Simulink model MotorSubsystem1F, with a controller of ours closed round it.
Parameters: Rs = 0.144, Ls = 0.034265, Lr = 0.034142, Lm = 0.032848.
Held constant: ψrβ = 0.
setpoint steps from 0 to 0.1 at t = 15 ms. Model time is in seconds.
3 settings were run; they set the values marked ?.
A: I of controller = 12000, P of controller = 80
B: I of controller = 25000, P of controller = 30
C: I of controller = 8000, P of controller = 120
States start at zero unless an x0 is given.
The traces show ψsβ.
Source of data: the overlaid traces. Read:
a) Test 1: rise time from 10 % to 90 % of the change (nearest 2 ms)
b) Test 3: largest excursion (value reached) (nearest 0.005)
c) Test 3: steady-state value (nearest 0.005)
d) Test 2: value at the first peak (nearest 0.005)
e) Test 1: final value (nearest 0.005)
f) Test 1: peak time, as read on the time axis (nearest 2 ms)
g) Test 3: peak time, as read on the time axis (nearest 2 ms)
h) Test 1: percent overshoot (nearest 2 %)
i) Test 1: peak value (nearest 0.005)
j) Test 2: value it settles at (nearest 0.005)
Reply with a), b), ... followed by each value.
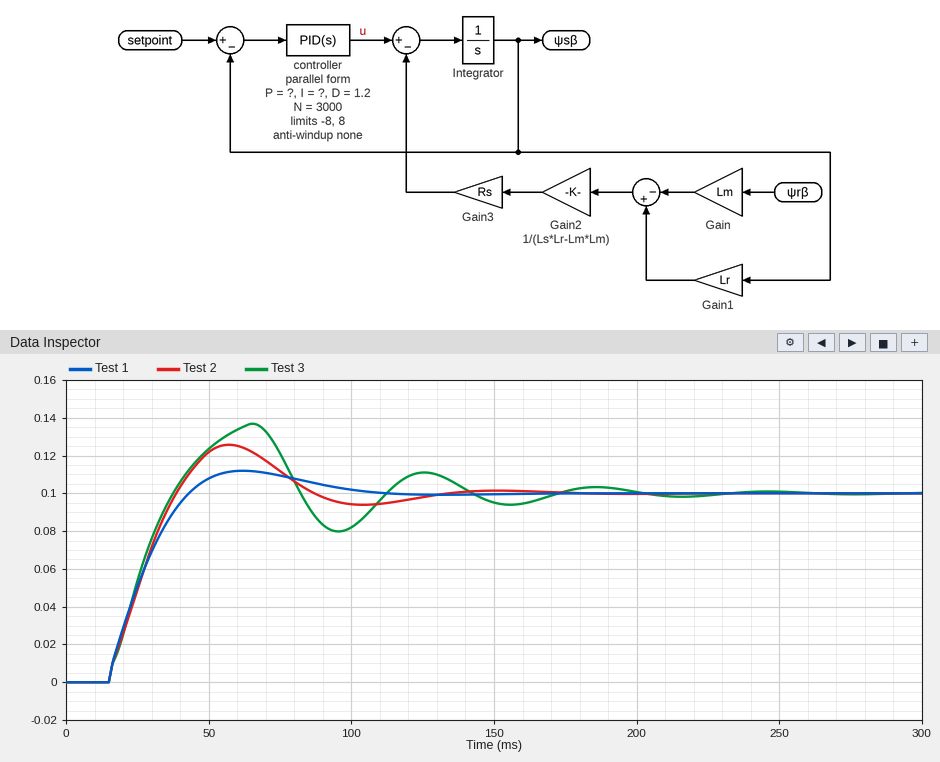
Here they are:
a) 22 ms
b) 0.135
c) 0.100
d) 0.125
e) 0.100
f) 62 ms
g) 66 ms
h) 12 %
i) 0.110
j) 0.100
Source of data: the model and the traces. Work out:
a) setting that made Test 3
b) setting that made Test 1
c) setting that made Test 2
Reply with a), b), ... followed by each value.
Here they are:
a) B
b) C
c) A
